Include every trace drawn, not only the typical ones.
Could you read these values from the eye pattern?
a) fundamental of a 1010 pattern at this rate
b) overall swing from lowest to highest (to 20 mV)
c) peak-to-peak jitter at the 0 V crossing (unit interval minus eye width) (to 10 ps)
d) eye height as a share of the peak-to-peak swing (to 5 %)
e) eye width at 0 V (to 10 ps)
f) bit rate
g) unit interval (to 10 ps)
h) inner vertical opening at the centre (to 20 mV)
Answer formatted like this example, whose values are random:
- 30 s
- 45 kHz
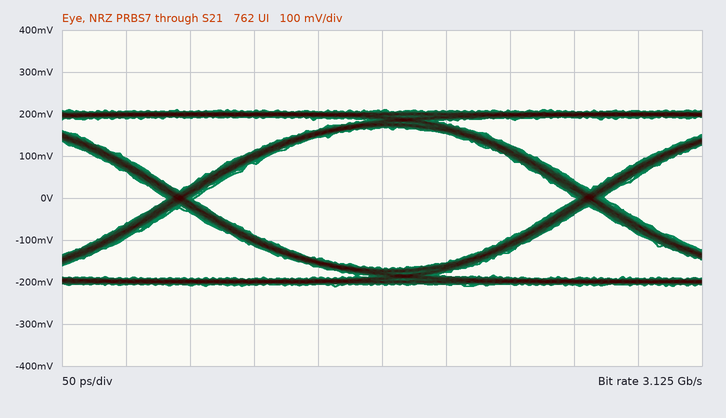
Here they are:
- 1.5625 GHz
- 420 mV
- 20 ps
- 80 %
- 300 ps
- 3.125 Gb/s
- 320 ps
- 340 mV
